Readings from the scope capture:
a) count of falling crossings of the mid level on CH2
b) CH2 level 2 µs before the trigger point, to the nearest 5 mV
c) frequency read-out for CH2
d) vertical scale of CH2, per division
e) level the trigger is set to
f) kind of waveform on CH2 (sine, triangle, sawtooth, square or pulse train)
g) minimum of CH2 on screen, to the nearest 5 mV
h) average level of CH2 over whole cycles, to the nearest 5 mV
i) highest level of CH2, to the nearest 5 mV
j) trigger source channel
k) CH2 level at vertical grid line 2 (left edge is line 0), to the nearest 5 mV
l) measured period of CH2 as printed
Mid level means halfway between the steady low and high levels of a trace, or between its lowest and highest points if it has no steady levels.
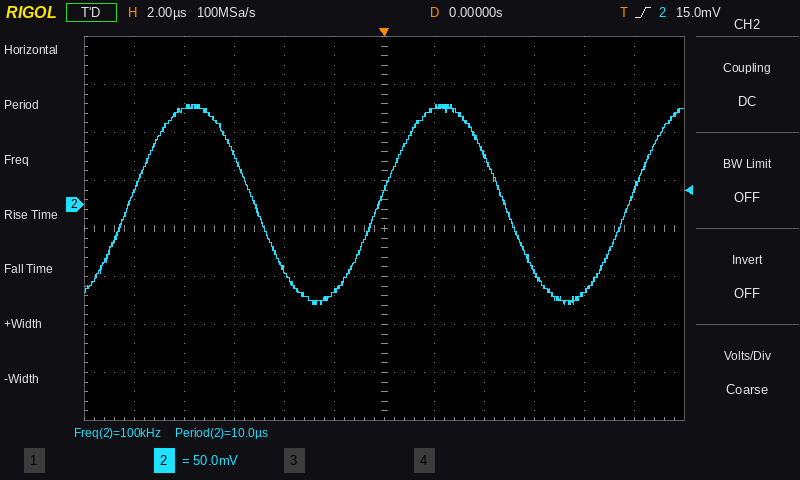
2
-90 mV
100 kHz
50 mV
15.0 mV
sine
-105 mV
0 mV
105 mV
CH2
100 mV
10.0 µs
